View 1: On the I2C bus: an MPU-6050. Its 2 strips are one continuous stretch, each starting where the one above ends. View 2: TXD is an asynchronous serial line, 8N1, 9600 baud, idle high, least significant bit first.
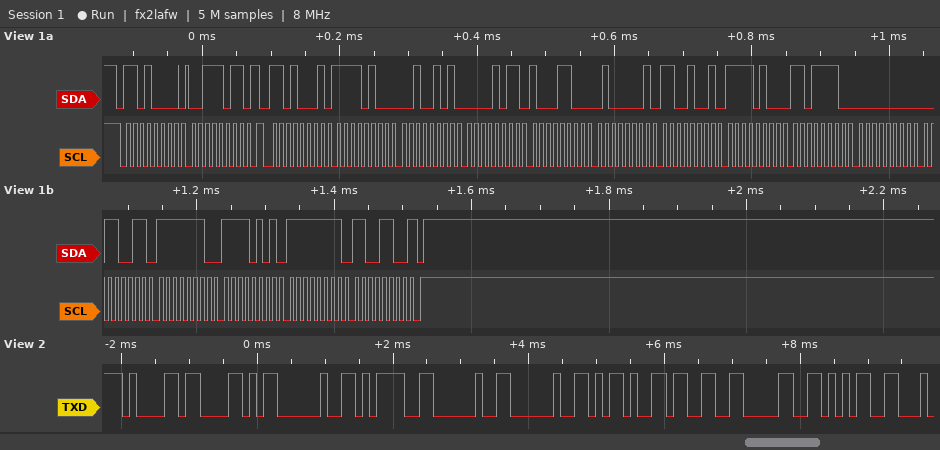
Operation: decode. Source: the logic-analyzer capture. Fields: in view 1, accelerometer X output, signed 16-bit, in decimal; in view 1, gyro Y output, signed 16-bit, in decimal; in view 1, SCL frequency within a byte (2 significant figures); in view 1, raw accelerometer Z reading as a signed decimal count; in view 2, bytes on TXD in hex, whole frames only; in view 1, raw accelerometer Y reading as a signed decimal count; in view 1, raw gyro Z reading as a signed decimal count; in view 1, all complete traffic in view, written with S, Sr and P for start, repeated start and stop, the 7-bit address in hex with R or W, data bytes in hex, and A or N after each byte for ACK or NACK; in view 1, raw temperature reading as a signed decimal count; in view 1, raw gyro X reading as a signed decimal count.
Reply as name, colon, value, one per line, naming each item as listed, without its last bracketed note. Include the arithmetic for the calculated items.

in view 1, accelerometer X output, signed 16-bit, in decimal: 0xF425 = -3035
in view 1, gyro Y output, signed 16-bit, in decimal: 0xFEF5 = -267
in view 1, SCL frequency within a byte: 100 kHz
in view 1, raw accelerometer Z reading as a signed decimal count: 0x41C9 = 16841
in view 2, bytes on TXD in hex, whole frames only: 0x61 0x58 0x20 0x3D 0x20 0x20 0x2D 0x33 0x30 0x35
in view 1, raw accelerometer Y reading as a signed decimal count: 0x0B8C = 2956
in view 1, raw gyro Z reading as a signed decimal count: 0xFFCC = -52
in view 1, all complete traffic in view, written with S, Sr and P for start, repeated start and stop, the 7-bit address in hex with R or W, data bytes in hex, and A or N after each byte for ACK or NACK: S 68W A 3B A Sr 68R A F4 A 25 A 0B A 8C A 41 A C9 A F4 A DE A 00 A 33 A FE A F5 A FF A CC N P
in view 1, raw temperature reading as a signed decimal count: 0xF4DE = -2850
in view 1, raw gyro X reading as a signed decimal count: 0x0033 = 51
